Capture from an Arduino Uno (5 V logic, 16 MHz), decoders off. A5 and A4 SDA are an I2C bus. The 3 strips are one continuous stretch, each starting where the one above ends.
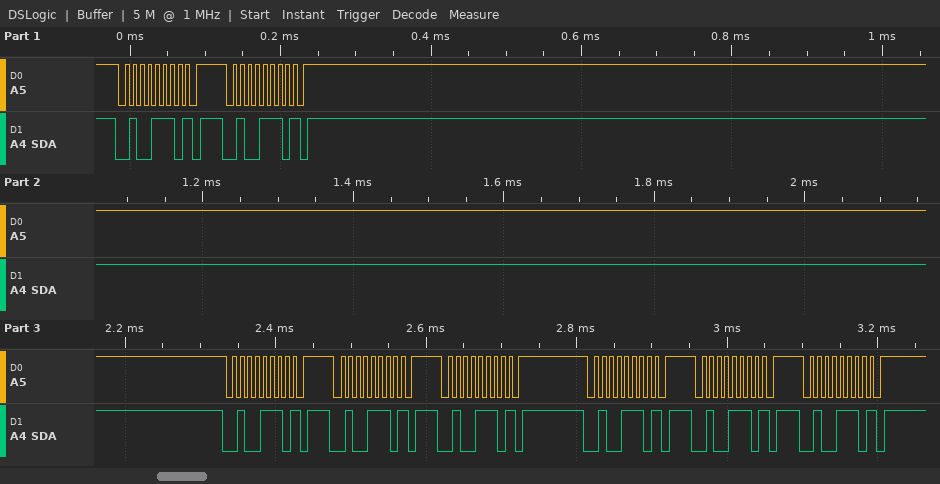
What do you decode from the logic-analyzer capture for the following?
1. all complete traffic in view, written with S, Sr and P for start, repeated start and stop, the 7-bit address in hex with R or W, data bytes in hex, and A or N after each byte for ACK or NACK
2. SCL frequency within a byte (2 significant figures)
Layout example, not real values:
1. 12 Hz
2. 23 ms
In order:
1. S 27W N P S 27W N P S 27W N P S 27W N P S 27W N P S 27W N P S 27W N P S 27W N P
2. 100 kHz
